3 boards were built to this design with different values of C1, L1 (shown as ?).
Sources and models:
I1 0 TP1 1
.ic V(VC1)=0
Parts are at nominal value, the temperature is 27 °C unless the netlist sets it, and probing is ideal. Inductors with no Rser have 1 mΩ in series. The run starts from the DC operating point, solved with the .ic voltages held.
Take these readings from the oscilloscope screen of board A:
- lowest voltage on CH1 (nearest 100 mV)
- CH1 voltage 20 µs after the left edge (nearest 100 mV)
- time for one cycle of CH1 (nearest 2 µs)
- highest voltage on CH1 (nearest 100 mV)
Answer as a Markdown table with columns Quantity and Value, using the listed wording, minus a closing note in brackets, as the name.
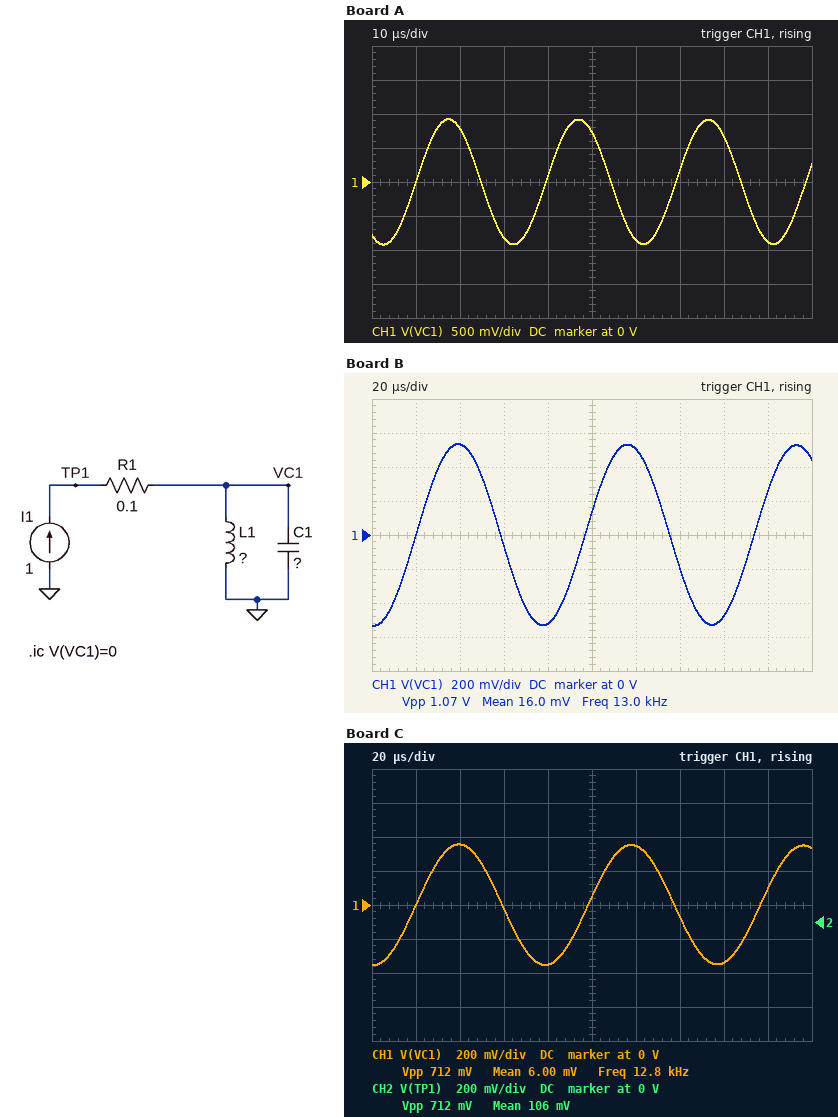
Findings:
| Quantity | Value |
|---|---|
| lowest voltage on CH1 | -900 mV |
| CH1 voltage 20 µs after the left edge | 800 mV |
| time for one cycle of CH1 | 30 µs |
| highest voltage on CH1 | 900 mV |
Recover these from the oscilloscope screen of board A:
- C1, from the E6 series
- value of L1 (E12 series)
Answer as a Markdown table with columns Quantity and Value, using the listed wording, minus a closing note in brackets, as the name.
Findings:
| Quantity | Value |
|---|---|
| C1, from the E6 series | 4.7 µF |
| value of L1 | 4.7 µH |
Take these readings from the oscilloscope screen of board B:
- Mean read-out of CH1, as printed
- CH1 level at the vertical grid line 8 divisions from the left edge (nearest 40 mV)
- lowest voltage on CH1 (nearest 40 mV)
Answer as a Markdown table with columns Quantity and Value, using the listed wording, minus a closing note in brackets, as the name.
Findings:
| Quantity | Value |
|---|---|
| Mean read-out of CH1, as printed | 16.0 mV |
| CH1 level at the vertical grid line 8 divisions from the left edge | -480 mV |
| lowest voltage on CH1 | -520 mV |
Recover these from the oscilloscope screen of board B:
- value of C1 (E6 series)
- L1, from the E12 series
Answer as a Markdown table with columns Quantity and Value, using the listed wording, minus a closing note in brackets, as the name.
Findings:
| Quantity | Value |
|---|---|
| value of C1 | 22 µF |
| L1, from the E12 series | 6.8 µH |
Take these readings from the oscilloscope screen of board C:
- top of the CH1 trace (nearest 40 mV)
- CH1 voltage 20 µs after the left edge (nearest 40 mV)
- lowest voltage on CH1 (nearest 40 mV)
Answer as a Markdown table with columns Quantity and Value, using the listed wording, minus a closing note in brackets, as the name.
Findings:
| Quantity | Value |
|---|---|
| top of the CH1 trace | 360 mV |
| CH1 voltage 20 µs after the left edge | 0 V |
| lowest voltage on CH1 | -360 mV |
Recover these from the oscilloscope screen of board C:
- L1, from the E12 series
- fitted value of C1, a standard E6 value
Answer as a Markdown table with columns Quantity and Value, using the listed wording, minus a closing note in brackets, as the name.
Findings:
| Quantity | Value |
|---|---|
| L1, from the E12 series | 4.7 µH |
| fitted value of C1, a standard E6 value | 33 µF |
